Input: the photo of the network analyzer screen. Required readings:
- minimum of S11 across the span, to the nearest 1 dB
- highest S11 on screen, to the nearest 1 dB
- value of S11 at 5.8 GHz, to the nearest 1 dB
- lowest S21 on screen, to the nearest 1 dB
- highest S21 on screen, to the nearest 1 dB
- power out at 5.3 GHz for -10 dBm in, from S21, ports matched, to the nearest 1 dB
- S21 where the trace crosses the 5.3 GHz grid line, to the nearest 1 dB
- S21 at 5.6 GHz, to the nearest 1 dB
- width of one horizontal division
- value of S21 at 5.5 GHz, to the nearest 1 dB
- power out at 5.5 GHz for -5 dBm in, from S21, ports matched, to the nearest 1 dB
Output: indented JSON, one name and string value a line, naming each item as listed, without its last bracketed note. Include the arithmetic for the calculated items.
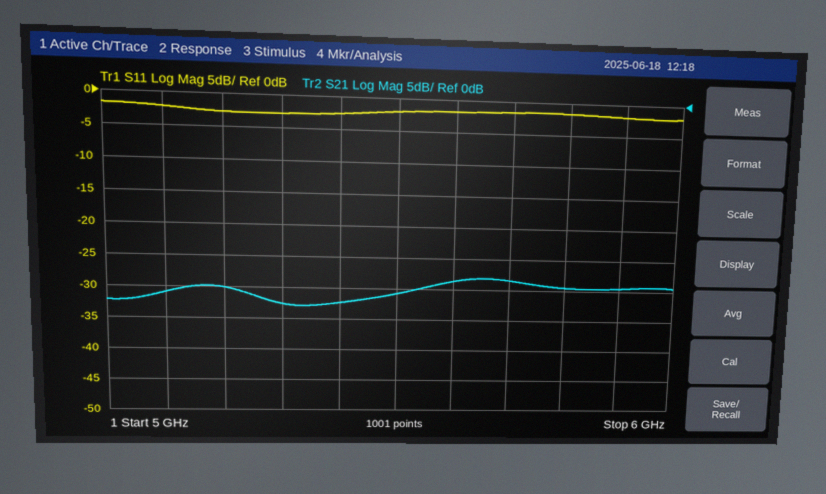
{
  "minimum of S11 across the span, to the nearest 1 dB": "-3 dB",
  "highest S11 on screen, to the nearest 1 dB": "-2 dB",
  "value of S11 at 5.8 GHz, to the nearest 1 dB": "-2 dB",
  "lowest S21 on screen, to the nearest 1 dB": "-33 dB",
  "highest S21 on screen, to the nearest 1 dB": "-28 dB",
  "power out at 5.3 GHz for -10 dBm in, from S21, ports matched, to the nearest 1 dB": "-10 dBm + (-33 dB) = -43 dBm",
  "S21 where the trace crosses the 5.3 GHz grid line, to the nearest 1 dB": "-33 dB",
  "S21 at 5.6 GHz, to the nearest 1 dB": "-29 dB",
  "width of one horizontal division": "100 MHz",
  "value of S21 at 5.5 GHz, to the nearest 1 dB": "-31 dB",
  "power out at 5.5 GHz for -5 dBm in, from S21, ports matched, to the nearest 1 dB": "-5 dBm + (-31 dB) = -36 dBm"
}
